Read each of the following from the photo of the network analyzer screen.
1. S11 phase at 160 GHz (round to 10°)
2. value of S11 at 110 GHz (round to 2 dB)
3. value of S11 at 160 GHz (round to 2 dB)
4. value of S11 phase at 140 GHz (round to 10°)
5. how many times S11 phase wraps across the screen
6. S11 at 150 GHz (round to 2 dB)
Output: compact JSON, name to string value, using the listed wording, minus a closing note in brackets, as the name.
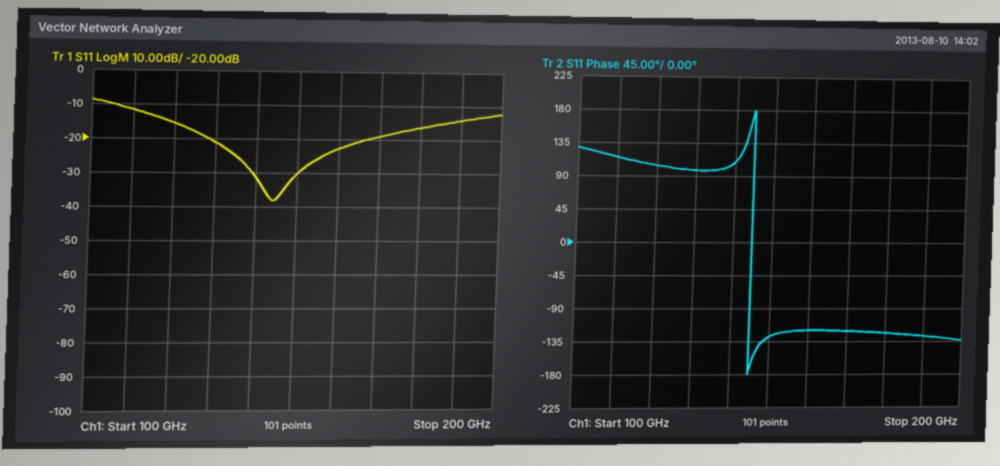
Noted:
{"S11 phase at 160 GHz": "-120°", "value of S11 at 110 GHz": "-12 dB", "value of S11 at 160 GHz": "-22 dB", "value of S11 phase at 140 GHz": "110°", "how many times S11 phase wraps across the screen": "1", "S11 at 150 GHz": "-30 dB"}
